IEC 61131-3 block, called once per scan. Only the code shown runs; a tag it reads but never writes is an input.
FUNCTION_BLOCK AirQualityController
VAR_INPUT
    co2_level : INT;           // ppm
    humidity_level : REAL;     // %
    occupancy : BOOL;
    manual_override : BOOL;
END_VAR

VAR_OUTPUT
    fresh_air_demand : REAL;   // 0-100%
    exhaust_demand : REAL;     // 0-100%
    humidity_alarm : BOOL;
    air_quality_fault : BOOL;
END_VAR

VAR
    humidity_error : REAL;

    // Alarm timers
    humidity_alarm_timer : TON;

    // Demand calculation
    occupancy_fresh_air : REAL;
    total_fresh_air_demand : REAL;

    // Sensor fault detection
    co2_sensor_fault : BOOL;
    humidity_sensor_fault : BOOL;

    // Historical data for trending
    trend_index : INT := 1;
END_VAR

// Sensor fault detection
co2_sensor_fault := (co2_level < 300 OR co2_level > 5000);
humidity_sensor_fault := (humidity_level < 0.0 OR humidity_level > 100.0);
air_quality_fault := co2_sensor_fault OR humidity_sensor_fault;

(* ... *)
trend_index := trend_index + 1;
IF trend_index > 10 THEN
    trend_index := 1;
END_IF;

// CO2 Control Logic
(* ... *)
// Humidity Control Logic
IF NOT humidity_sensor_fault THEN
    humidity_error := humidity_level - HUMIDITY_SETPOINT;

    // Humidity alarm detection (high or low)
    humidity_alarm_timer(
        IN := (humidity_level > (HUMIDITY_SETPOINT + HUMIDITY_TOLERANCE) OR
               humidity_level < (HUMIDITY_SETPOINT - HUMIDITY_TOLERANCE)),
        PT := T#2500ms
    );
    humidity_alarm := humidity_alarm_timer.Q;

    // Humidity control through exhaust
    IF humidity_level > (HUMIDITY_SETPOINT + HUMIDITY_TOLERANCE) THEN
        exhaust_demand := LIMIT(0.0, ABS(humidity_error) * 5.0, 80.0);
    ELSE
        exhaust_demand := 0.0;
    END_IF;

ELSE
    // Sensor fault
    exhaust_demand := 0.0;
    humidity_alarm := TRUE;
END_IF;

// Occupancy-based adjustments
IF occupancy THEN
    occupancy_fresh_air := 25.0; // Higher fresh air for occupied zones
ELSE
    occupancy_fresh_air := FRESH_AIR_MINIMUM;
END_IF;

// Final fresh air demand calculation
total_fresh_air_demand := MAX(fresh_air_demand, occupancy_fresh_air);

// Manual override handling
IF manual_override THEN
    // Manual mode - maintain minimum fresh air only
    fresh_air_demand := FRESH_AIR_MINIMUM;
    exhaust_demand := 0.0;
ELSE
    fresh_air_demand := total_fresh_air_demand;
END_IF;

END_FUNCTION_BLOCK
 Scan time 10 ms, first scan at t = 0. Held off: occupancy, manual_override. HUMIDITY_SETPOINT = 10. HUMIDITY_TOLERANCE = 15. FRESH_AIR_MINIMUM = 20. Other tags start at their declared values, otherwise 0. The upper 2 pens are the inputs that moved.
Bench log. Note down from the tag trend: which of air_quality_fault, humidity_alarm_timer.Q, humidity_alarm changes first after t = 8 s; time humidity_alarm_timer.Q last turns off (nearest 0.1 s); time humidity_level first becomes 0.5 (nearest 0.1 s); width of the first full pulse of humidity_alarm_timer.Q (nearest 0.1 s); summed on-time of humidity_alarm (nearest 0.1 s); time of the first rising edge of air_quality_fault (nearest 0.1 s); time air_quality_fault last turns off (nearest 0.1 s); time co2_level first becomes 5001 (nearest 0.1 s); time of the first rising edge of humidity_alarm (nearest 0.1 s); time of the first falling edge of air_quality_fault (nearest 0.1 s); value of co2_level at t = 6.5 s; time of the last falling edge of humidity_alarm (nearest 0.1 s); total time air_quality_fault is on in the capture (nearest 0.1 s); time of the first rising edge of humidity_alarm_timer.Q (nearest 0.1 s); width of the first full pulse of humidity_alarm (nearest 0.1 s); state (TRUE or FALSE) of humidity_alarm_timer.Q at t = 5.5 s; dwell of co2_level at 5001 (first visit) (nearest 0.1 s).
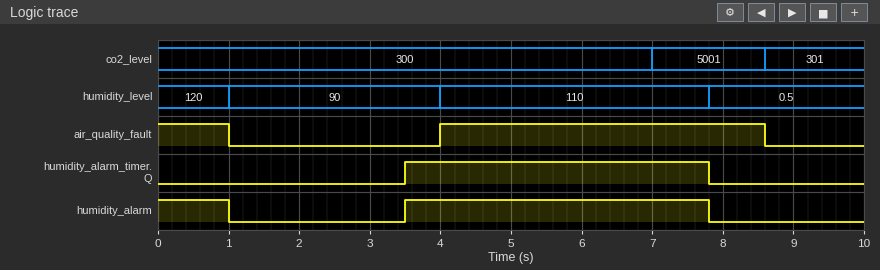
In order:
air_quality_fault
7.8 s
7.8 s
4.3 s
5.3 s
4.0 s
8.6 s
7.0 s
3.5 s
1.0 s
300
7.8 s
5.6 s
3.5 s
4.3 s
TRUE
1.6 s
